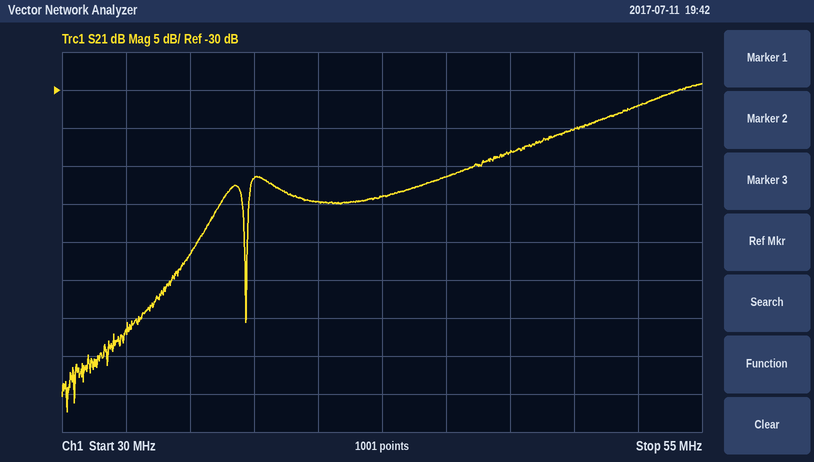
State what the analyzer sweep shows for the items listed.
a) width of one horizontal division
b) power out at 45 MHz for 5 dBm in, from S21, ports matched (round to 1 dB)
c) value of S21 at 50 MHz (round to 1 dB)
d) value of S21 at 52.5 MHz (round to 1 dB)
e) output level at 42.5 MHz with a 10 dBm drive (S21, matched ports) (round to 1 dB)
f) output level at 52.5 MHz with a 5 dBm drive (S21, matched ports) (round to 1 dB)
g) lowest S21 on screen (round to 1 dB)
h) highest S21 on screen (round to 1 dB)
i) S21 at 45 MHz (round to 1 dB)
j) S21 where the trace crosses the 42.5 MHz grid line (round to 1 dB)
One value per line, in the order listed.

2.5 MHz
-36 dBm
-35 dB
-32 dB
-34 dBm
-27 dBm
-72 dB
-29 dB
-41 dB
-44 dB
